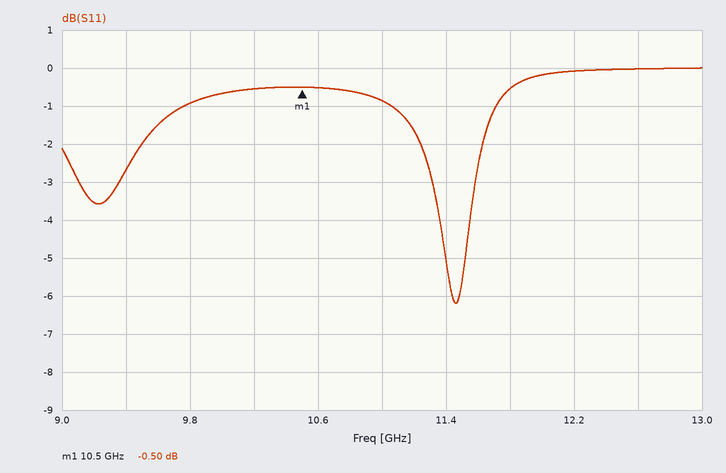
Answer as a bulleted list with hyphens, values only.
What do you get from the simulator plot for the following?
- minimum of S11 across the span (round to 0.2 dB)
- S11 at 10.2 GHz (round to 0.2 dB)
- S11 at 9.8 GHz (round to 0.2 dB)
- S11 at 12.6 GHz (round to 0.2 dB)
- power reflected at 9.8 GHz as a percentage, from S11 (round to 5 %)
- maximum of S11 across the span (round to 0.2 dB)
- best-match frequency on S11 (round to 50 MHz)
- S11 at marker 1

- -6.2 dB
- -0.6 dB
- -1.0 dB
- 0.0 dB
- 80 %
- 0.0 dB
- 11.45 GHz
- -0.50 dB
